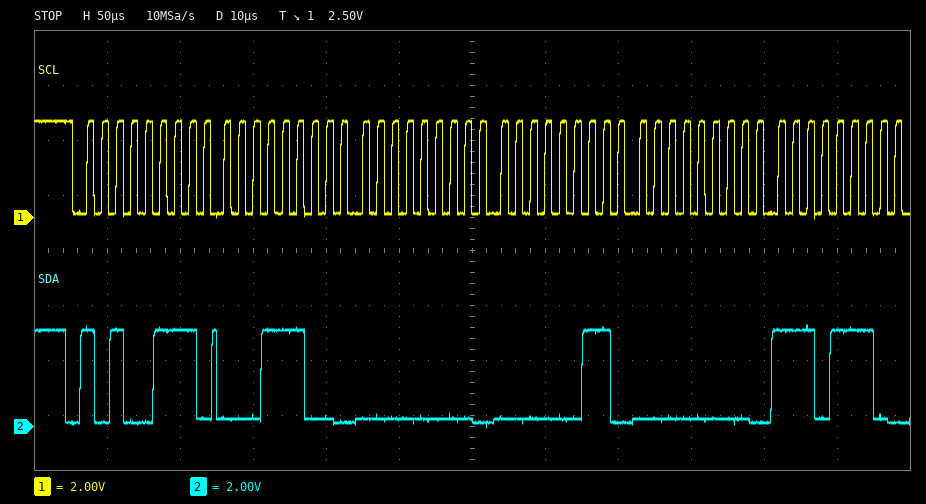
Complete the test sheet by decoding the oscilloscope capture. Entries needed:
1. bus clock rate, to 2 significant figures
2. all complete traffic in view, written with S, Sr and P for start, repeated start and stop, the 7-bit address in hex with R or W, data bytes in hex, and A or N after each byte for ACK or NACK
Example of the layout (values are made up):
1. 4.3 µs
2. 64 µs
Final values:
1. 100 kHz
2. S 53R A 1C A 00 A 03 A 00 A EE A
